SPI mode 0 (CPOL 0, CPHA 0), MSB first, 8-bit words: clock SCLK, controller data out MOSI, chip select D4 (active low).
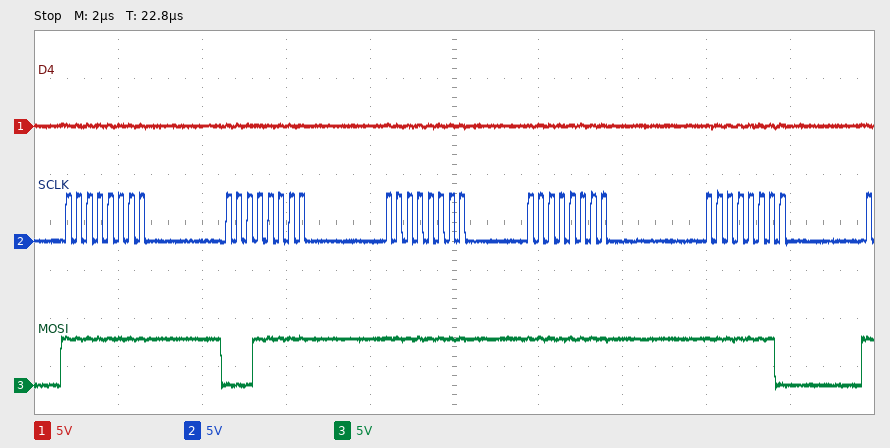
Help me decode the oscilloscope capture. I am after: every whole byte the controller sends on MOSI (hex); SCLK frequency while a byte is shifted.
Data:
FF 1F FF FF FE
4 MHz
